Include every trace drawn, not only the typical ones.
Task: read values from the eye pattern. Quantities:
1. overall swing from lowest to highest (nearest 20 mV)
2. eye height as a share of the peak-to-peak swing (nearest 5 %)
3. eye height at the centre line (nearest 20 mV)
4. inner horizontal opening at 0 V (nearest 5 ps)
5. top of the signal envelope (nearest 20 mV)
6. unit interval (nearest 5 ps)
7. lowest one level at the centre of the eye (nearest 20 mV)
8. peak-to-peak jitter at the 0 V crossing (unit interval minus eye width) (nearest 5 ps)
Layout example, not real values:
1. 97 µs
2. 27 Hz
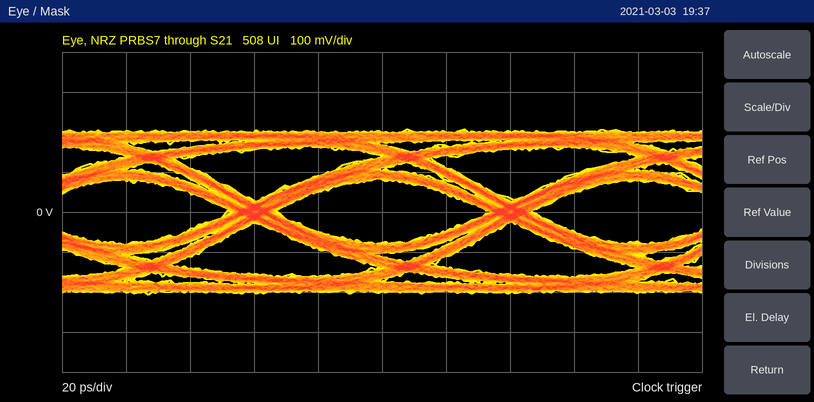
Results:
1. 420 mV
2. 40 %
3. 160 mV
4. 65 ps
5. 200 mV
6. 80 ps
7. 80 mV
8. 15 ps
